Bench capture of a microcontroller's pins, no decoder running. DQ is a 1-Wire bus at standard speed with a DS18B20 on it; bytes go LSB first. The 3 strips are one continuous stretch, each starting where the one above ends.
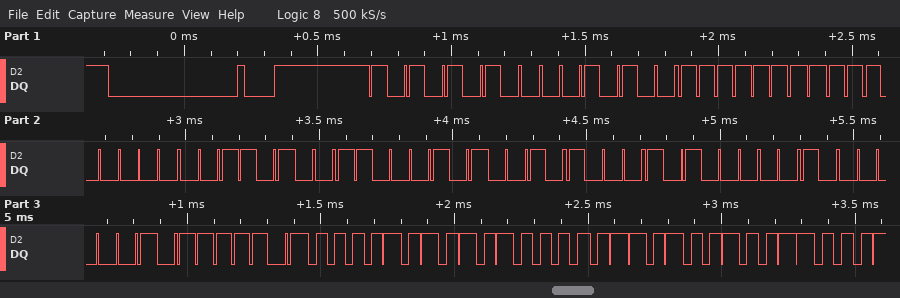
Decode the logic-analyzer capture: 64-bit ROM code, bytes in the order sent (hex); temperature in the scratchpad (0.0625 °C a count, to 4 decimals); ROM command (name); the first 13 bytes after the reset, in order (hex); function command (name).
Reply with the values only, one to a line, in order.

28 FF 07 2C A3 14 05 81
85.0000 °C
Match ROM
55 28 FF 07 2C A3 14 05 81 BE 50 05 4B
Read Scratchpad
